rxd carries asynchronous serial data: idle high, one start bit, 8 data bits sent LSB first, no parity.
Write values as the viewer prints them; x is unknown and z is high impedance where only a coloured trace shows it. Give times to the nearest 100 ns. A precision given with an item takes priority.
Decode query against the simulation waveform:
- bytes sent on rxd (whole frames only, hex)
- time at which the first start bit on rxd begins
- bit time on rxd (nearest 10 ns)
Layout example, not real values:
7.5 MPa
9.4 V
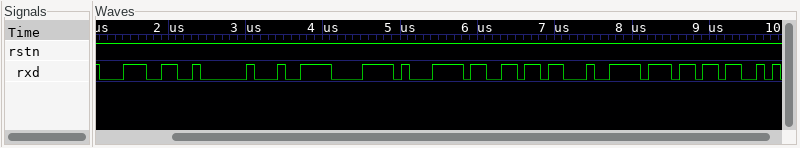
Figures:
9C, 02, E4, 78, BC, B6, E4, B7
1100 ns
100 ns
